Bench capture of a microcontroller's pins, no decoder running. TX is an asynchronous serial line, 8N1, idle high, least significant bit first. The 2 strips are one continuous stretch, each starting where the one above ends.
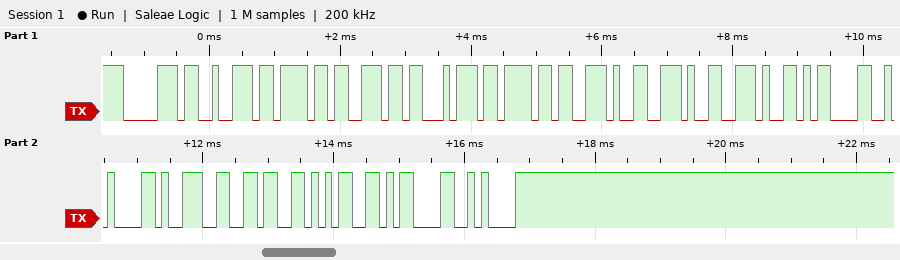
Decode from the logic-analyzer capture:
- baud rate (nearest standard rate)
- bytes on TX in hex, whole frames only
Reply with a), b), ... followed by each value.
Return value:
a) 9600 baud
b) 70 72 6F 6E 74 6F 2E 2E 2E 0D 0A 39 36 35 0D 0A
